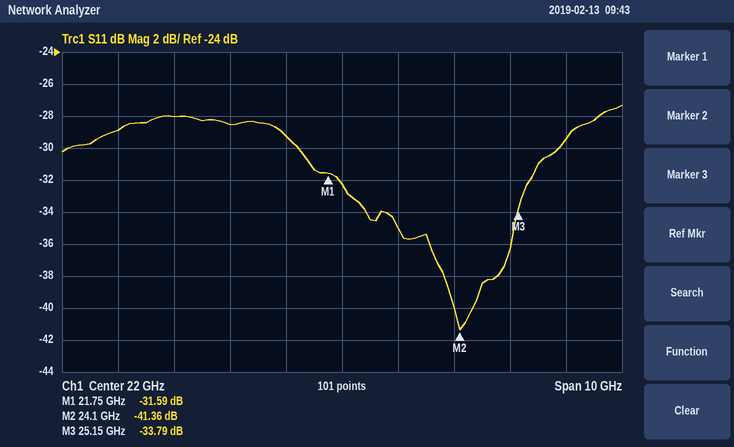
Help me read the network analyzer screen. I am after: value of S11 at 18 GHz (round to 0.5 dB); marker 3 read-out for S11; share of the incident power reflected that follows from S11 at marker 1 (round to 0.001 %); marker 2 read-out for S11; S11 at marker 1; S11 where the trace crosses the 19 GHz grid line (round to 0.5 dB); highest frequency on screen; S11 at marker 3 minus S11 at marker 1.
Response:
-29.0 dB
-33.79 dB
0.069 %
-41.36 dB
-31.59 dB
-28.0 dB
27 GHz
-2.20 dB
